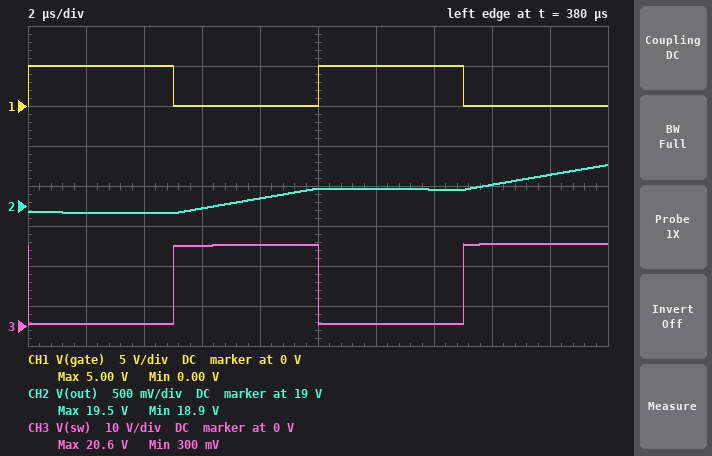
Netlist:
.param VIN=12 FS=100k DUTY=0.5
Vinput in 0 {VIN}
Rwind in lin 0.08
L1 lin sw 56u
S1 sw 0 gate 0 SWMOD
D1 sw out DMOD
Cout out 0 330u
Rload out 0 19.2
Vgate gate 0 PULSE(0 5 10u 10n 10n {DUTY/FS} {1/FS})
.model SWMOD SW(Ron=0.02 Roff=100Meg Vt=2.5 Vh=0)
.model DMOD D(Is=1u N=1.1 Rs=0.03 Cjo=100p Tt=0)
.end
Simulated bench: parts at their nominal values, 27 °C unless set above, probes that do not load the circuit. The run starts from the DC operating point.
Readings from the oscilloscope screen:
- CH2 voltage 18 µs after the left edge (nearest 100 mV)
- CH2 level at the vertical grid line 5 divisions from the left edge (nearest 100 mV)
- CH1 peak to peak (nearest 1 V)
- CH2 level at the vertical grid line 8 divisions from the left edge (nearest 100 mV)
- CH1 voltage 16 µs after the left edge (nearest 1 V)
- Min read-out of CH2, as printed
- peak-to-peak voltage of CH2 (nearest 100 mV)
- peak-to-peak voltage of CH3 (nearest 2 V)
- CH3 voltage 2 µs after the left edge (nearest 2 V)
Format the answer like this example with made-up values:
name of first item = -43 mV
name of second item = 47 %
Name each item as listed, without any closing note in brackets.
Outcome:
CH2 voltage 18 µs after the left edge = 19.4 V
CH2 level at the vertical grid line 5 divisions from the left edge = 19.2 V
CH1 peak to peak = 5 V
CH2 level at the vertical grid line 8 divisions from the left edge = 19.3 V
CH1 voltage 16 µs after the left edge = 0 V
Min read-out of CH2, as printed = 18.9 V
peak-to-peak voltage of CH2 = 600 mV
peak-to-peak voltage of CH3 = 20 V
CH3 voltage 2 µs after the left edge = 0 V
